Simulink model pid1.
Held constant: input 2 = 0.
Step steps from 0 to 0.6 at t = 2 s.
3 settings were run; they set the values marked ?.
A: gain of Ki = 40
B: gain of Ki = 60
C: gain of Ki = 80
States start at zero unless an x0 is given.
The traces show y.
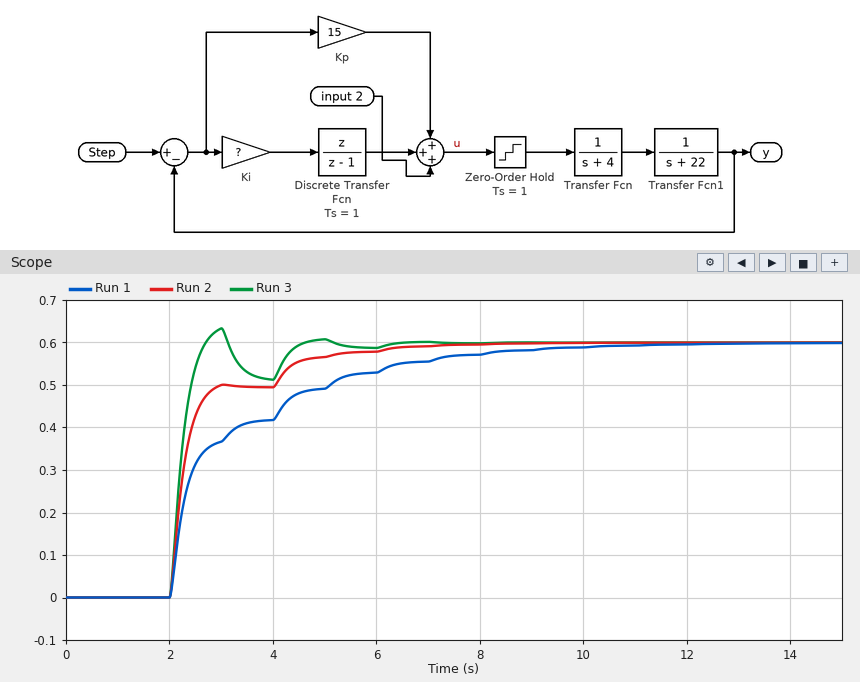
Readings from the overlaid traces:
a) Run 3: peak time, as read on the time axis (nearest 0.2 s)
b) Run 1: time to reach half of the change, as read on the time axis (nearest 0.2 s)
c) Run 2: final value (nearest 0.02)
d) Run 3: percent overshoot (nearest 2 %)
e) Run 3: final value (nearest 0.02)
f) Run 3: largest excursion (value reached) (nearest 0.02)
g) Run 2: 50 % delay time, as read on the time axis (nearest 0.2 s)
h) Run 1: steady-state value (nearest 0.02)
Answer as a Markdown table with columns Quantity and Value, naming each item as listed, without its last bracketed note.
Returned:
| Quantity | Value |
|---|---|
| Run 3: peak time, as read on the time axis | 3.0 s |
| Run 1: time to reach half of the change, as read on the time axis | 2.4 s |
| Run 2: final value | 0.60 |
| Run 3: percent overshoot | 6 % |
| Run 3: final value | 0.60 |
| Run 3: largest excursion (value reached) | 0.64 |
| Run 2: 50 % delay time, as read on the time axis | 2.2 s |
| Run 1: steady-state value | 0.60 |
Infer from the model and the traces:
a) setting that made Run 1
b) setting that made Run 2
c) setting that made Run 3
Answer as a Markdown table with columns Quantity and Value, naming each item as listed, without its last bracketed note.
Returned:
| Quantity | Value |
|---|---|
| setting that made Run 1 | A |
| setting that made Run 2 | B |
| setting that made Run 3 | C |
